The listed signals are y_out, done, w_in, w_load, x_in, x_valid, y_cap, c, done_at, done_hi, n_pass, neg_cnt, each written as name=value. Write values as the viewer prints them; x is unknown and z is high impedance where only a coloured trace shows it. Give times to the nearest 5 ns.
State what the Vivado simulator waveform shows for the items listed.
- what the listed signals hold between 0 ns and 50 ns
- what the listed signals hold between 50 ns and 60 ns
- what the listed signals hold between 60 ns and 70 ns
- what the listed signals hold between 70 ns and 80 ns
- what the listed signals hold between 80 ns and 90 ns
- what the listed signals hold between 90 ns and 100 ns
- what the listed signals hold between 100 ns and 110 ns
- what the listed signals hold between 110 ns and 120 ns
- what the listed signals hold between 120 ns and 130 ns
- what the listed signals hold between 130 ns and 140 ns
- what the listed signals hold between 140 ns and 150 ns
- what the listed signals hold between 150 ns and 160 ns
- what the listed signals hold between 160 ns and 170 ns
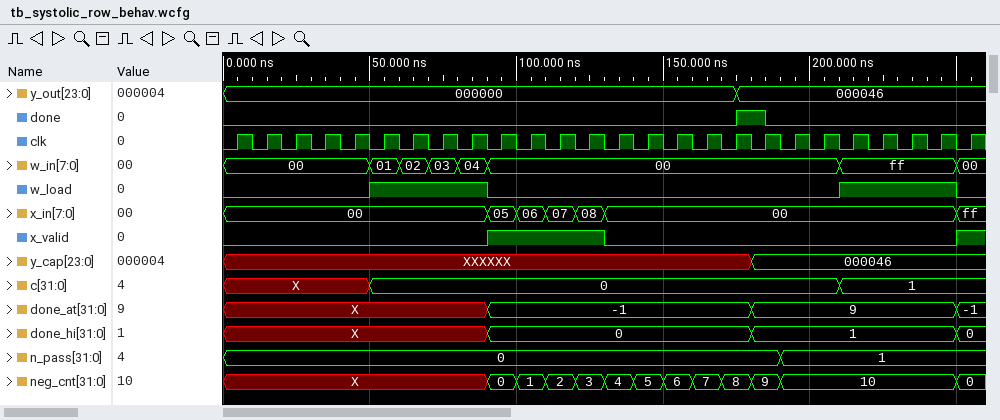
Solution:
y_out=000000, done=0, w_in=00, w_load=0, x_in=00, x_valid=0, y_cap=XXXXXX, c=X, done_at=X, done_hi=X, n_pass=0, neg_cnt=X
y_out=000000, done=0, w_in=01, w_load=1, x_in=00, x_valid=0, y_cap=XXXXXX, c=0, done_at=X, done_hi=X, n_pass=0, neg_cnt=X
y_out=000000, done=0, w_in=02, w_load=1, x_in=00, x_valid=0, y_cap=XXXXXX, c=0, done_at=X, done_hi=X, n_pass=0, neg_cnt=X
y_out=000000, done=0, w_in=03, w_load=1, x_in=00, x_valid=0, y_cap=XXXXXX, c=0, done_at=X, done_hi=X, n_pass=0, neg_cnt=X
y_out=000000, done=0, w_in=04, w_load=1, x_in=00, x_valid=0, y_cap=XXXXXX, c=0, done_at=X, done_hi=X, n_pass=0, neg_cnt=X
y_out=000000, done=0, w_in=00, w_load=0, x_in=05, x_valid=1, y_cap=XXXXXX, c=0, done_at=-1, done_hi=0, n_pass=0, neg_cnt=0
y_out=000000, done=0, w_in=00, w_load=0, x_in=06, x_valid=1, y_cap=XXXXXX, c=0, done_at=-1, done_hi=0, n_pass=0, neg_cnt=1
y_out=000000, done=0, w_in=00, w_load=0, x_in=07, x_valid=1, y_cap=XXXXXX, c=0, done_at=-1, done_hi=0, n_pass=0, neg_cnt=2
y_out=000000, done=0, w_in=00, w_load=0, x_in=08, x_valid=1, y_cap=XXXXXX, c=0, done_at=-1, done_hi=0, n_pass=0, neg_cnt=3
y_out=000000, done=0, w_in=00, w_load=0, x_in=00, x_valid=0, y_cap=XXXXXX, c=0, done_at=-1, done_hi=0, n_pass=0, neg_cnt=4
y_out=000000, done=0, w_in=00, w_load=0, x_in=00, x_valid=0, y_cap=XXXXXX, c=0, done_at=-1, done_hi=0, n_pass=0, neg_cnt=5
y_out=000000, done=0, w_in=00, w_load=0, x_in=00, x_valid=0, y_cap=XXXXXX, c=0, done_at=-1, done_hi=0, n_pass=0, neg_cnt=6
y_out=000000, done=0, w_in=00, w_load=0, x_in=00, x_valid=0, y_cap=XXXXXX, c=0, done_at=-1, done_hi=0, n_pass=0, neg_cnt=7
